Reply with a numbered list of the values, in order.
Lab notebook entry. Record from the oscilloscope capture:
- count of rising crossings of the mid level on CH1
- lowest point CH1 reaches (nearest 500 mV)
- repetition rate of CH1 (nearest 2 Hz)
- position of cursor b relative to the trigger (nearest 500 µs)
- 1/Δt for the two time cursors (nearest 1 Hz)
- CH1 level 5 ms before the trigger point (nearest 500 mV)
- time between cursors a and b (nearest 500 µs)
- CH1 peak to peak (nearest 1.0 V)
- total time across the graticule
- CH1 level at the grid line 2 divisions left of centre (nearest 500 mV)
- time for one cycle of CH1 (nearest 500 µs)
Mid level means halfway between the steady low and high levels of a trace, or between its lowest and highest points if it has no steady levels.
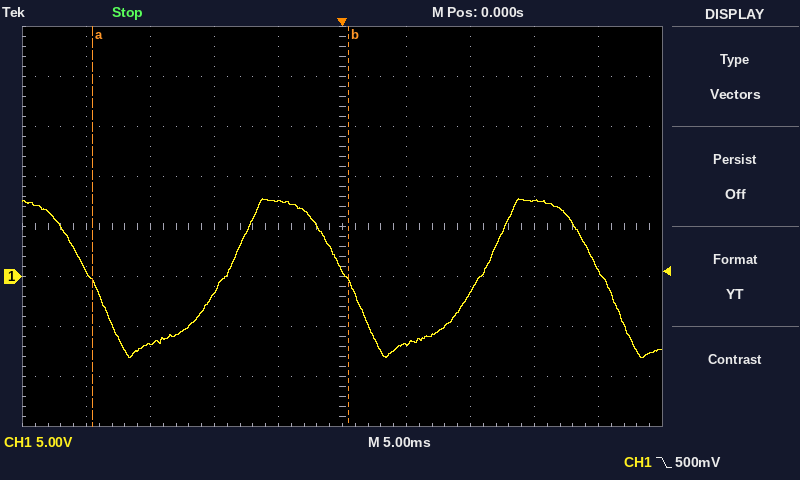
1. 2
2. -8.0 V
3. 50 Hz
4. +500 µs
5. 50 Hz
6. 7.5 V
7. 20.0 ms
8. 16.0 V
9. 50 ms
10. -1.5 V
11. 20.0 ms
